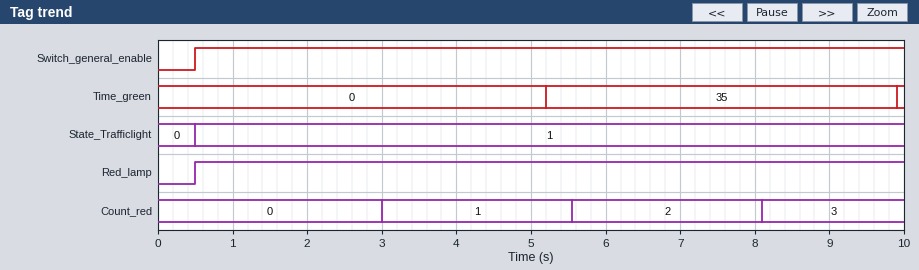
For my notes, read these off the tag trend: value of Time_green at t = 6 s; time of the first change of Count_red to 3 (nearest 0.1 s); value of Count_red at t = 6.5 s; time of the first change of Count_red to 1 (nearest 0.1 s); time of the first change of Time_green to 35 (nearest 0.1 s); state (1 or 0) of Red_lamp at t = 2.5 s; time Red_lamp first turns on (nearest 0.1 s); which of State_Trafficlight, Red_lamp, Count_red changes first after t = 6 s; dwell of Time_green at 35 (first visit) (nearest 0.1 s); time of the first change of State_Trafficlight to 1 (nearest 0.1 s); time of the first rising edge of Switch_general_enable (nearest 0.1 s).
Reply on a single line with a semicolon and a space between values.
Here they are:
35; 8.1 s; 2; 3.0 s; 5.2 s; 1; 0.5 s; Count_red; 4.7 s; 0.5 s; 0.5 s
